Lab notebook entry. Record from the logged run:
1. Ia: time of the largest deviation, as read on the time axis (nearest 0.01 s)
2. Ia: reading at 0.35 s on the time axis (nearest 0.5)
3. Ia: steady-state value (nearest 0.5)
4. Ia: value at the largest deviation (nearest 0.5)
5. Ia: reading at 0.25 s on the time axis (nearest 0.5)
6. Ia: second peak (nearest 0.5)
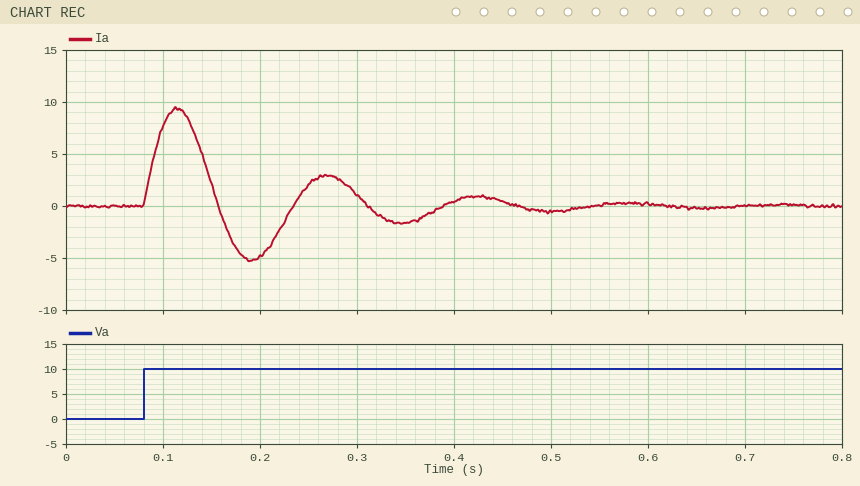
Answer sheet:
0.11 s
-1.5
0.0
9.5
2.0
3.0
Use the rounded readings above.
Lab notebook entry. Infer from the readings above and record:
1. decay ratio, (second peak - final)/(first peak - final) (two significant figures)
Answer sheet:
0.32
